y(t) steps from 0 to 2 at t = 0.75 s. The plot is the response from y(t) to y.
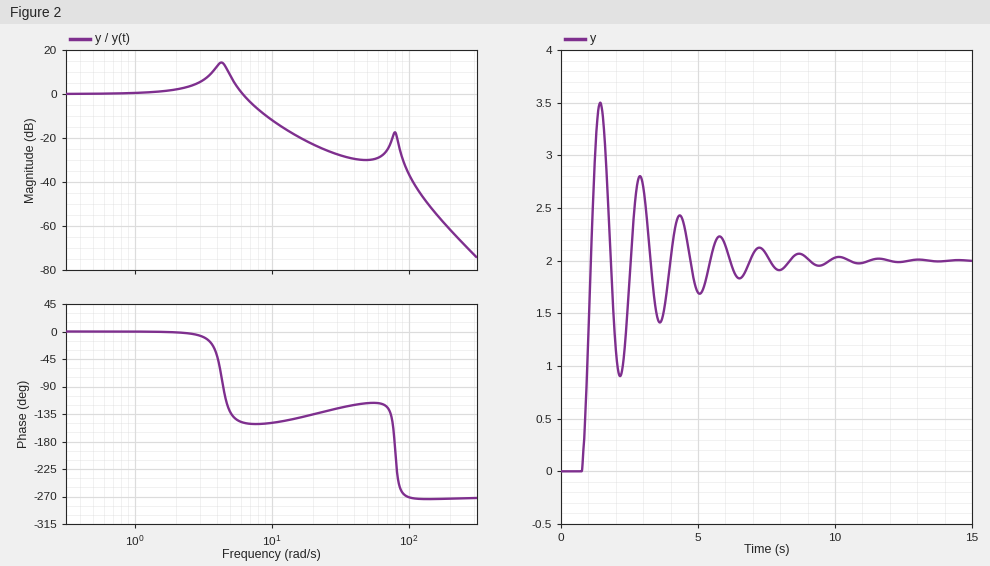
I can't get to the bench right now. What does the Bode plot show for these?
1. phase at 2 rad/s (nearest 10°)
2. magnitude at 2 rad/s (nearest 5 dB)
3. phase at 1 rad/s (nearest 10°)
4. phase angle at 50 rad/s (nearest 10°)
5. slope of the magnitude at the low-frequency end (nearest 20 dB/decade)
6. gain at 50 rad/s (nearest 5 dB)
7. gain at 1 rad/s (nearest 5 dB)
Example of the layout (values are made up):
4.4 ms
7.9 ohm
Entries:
0°
0 dB
0°
-120°
0 dB/decade
-30 dB
0 dB
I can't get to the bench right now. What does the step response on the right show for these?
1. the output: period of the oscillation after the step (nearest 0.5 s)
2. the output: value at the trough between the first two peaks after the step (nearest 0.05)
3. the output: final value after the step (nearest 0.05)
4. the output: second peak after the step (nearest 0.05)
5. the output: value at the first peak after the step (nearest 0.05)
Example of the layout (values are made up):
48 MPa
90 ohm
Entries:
1.5 s
0.90
2.00
2.80
3.50
